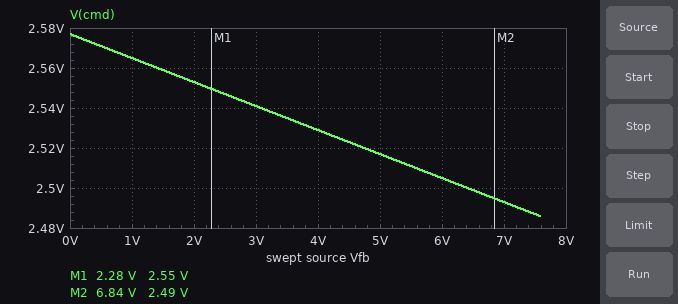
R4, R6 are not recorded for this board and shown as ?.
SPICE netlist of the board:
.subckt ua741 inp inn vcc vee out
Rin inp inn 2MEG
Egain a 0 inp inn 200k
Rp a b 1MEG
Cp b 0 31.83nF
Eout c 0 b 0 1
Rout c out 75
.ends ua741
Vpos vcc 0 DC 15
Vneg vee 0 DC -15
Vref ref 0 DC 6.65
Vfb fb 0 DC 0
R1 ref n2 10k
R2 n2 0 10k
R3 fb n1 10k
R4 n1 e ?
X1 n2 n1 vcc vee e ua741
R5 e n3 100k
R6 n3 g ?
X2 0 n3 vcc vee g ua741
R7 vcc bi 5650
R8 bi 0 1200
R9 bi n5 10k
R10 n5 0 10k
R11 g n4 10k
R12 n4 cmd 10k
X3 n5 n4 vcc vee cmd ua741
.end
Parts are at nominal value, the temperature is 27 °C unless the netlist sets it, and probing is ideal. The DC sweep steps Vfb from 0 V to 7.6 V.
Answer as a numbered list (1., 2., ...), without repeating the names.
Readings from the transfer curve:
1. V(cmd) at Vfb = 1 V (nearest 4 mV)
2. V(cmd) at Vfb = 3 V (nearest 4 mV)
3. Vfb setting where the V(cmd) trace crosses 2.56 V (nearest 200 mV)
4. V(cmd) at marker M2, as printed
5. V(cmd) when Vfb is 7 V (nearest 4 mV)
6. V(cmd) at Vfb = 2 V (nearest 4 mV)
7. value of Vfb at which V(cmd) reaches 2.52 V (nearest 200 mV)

1. 2.564 V
2. 2.540 V
3. 1.4 V
4. 2.49 V
5. 2.492 V
6. 2.552 V
7. 4.8 V
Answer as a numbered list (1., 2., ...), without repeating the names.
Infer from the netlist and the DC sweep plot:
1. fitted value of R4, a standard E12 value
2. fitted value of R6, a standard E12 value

1. 12 kΩ
2. 1 kΩ
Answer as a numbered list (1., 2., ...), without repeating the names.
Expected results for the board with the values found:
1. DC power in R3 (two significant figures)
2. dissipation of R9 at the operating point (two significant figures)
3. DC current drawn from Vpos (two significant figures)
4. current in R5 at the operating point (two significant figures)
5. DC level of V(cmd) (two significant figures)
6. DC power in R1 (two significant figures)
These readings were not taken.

1. 1.1 mW
2. 160 µW
3. 2.2 mA
4. 73 µA
5. 2.6 V
6. 1.1 mW
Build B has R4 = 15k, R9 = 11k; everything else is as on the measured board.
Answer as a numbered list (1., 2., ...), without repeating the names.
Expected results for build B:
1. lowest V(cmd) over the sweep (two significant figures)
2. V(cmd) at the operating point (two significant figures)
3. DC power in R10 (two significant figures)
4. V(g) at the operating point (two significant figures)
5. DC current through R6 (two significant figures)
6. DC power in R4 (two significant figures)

1. 2.4 V
2. 2.5 V
3. 140 µW
4. -83 mV
5. 83 µA
6. 1.7 mW
